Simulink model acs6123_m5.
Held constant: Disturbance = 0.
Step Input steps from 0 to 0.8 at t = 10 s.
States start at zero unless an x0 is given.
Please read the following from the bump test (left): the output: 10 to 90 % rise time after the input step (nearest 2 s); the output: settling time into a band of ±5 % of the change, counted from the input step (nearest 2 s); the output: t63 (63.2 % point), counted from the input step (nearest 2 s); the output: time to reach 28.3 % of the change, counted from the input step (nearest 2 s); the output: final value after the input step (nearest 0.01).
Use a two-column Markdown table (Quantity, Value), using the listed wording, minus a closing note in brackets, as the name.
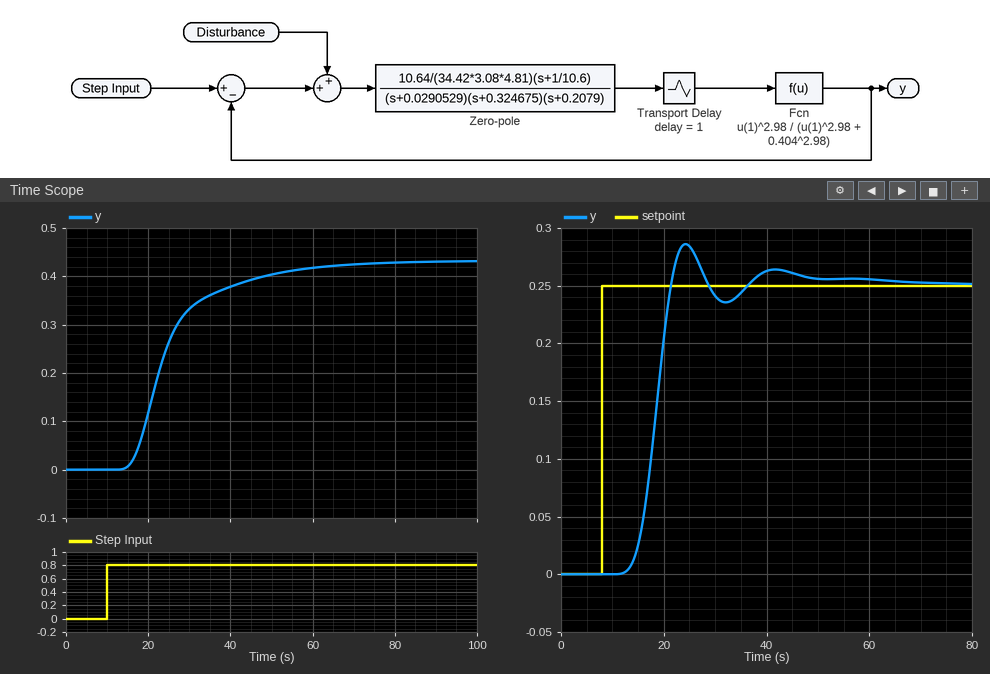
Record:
| Quantity | Value |
|---|---|
| the output: 10 to 90 % rise time after the input step | 26 s |
| the output: settling time into a band of ±5 % of the change, counted from the input step | 44 s |
| the output: t63 (63.2 % point), counted from the input step | 16 s |
| the output: time to reach 28.3 % of the change, counted from the input step | 10 s |
| the output: final value after the input step | 0.43 |
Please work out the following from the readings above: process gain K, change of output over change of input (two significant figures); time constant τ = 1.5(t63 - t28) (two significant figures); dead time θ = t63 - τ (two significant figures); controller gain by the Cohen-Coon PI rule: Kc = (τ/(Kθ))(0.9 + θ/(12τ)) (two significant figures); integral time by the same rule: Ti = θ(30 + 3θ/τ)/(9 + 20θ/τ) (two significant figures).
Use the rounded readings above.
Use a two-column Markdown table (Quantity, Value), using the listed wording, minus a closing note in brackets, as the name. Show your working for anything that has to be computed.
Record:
| Quantity | Value |
|---|---|
| process gain K, change of output over change of input | (0.43 - 0) / 0.8 = 0.54 |
| time constant τ = 1.5(t63 - t28) | 1.5 × (16 - 10) = 9.0 s |
| dead time θ = t63 - τ | 16 - 9 = 7.0 s |
| controller gain by the Cohen-Coon PI rule: Kc = (τ/(Kθ))(0.9 + θ/(12τ)) | 9 / (0.54 × 7) × (0.9 + 7 / (12 × 9)) = 2.3 |
| integral time by the same rule: Ti = θ(30 + 3θ/τ)/(9 + 20θ/τ) | 7 × (30 + 3 × 7 / 9) / (9 + 20 × 7 / 9) = 9.2 s |
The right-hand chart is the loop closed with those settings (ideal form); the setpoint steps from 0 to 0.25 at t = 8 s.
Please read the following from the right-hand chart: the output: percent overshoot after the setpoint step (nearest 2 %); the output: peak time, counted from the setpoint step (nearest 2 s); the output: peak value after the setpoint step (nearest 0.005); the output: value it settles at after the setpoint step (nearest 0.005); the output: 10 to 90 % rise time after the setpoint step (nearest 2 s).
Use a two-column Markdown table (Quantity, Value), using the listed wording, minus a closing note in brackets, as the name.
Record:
| Quantity | Value |
|---|---|
| the output: percent overshoot after the setpoint step | 14 % |
| the output: peak time, counted from the setpoint step | 16 s |
| the output: peak value after the setpoint step | 0.285 |
| the output: value it settles at after the setpoint step | 0.250 |
| the output: 10 to 90 % rise time after the setpoint step | 6 s |
